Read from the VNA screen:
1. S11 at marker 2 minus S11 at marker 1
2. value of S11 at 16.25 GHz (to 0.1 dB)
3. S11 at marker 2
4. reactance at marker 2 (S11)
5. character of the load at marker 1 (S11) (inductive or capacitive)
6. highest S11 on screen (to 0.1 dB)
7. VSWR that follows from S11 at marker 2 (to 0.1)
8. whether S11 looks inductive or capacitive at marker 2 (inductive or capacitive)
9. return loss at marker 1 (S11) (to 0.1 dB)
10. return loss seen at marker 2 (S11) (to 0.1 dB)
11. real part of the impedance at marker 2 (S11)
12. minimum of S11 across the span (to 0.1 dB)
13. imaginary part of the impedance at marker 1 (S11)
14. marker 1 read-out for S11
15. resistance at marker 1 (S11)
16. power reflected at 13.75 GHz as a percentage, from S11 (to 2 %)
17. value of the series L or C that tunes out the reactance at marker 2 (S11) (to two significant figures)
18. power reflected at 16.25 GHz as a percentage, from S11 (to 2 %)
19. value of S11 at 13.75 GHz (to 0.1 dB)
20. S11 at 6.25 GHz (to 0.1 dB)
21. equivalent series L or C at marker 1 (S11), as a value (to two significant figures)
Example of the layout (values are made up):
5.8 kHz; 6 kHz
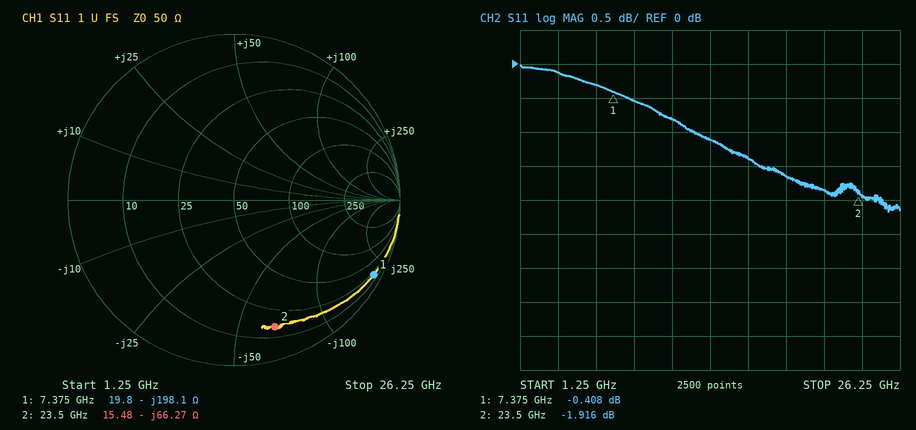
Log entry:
-1.508 dB; -1.4 dB; -1.916 dB; -66.27 Ω; capacitive; 0.0 dB; 9.1; capacitive; 0.4 dB; 1.9 dB; 15.48 Ω; -2.2 dB; -198.1 Ω; -0.408 dB; 19.8 Ω; 78 %; 450 pH; 72 %; -1.1 dB; -0.3 dB; 110 fF
